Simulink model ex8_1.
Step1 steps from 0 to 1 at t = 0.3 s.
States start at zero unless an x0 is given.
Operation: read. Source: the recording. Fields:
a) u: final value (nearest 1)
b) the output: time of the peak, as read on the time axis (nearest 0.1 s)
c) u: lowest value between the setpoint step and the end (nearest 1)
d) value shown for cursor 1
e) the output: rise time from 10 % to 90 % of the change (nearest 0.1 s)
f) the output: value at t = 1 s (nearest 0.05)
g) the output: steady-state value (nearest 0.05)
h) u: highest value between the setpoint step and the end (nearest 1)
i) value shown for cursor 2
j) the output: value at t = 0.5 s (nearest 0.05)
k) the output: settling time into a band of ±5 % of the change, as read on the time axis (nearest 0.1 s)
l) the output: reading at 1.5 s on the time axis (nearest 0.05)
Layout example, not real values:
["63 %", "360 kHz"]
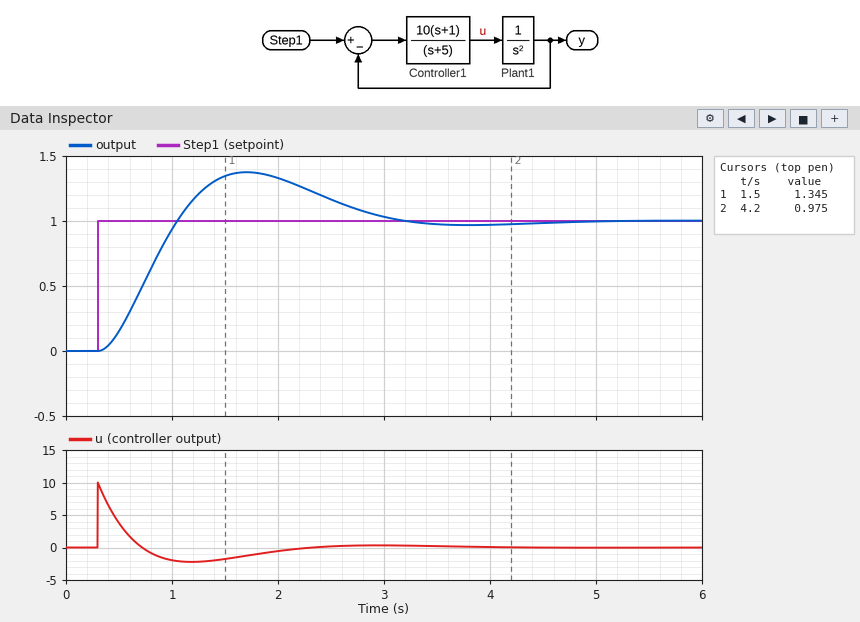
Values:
["0", "1.7 s", "-2", "1.345", "0.5 s", "0.95", "1.00", "10", "0.975", "0.15", "2.9 s", "1.35"]
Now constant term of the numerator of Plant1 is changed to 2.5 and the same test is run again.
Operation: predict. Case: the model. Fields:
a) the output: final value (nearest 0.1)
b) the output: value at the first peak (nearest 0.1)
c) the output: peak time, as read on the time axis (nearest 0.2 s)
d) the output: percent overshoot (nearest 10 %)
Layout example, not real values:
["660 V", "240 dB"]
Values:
["1.0", "1.4", "1.0 s", "40 %"]
